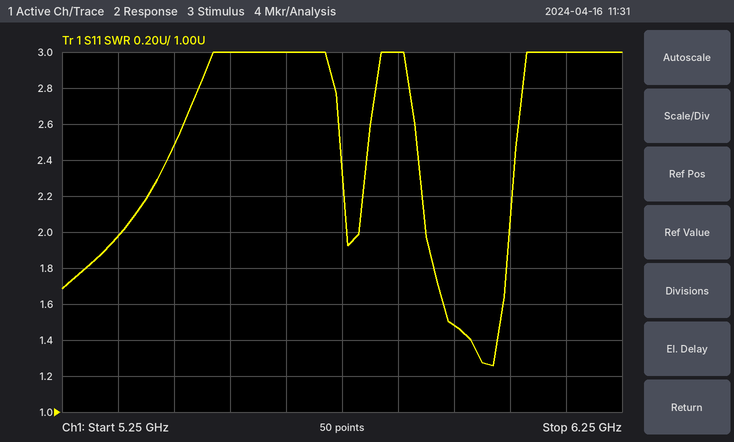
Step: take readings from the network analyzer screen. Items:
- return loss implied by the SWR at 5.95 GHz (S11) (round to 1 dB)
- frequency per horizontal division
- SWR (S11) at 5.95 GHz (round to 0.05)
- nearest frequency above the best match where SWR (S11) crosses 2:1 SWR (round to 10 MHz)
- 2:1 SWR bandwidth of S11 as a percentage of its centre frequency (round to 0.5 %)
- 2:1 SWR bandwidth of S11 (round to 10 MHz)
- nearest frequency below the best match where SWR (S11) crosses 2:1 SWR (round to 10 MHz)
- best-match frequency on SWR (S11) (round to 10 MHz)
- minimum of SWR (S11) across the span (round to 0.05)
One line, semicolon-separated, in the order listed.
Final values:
14 dB; 100 MHz; 1.50; 6.05 GHz; 2.5 %; 150 MHz; 5.90 GHz; 6.02 GHz; 1.25
